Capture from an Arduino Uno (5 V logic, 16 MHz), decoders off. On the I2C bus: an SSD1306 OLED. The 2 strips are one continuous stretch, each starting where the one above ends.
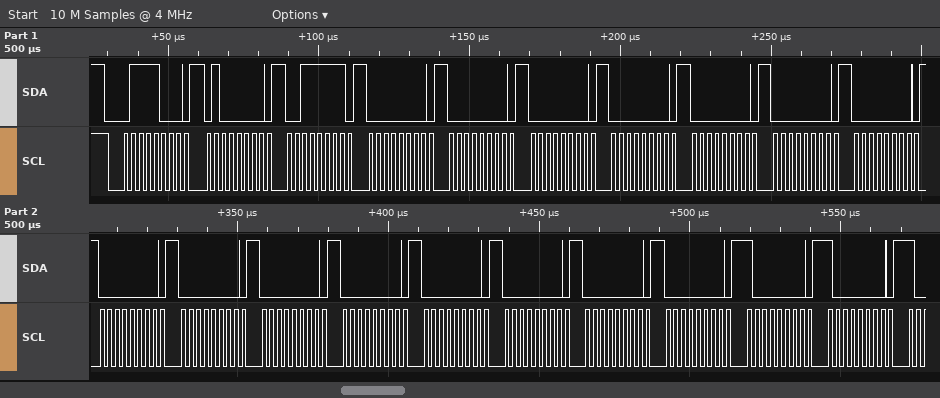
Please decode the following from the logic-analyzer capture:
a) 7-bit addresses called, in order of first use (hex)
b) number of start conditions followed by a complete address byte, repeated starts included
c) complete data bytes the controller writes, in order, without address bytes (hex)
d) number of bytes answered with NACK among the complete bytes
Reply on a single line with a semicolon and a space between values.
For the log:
0x3C; 1; 40 3F 00 00 00 00 00 00 00 00 00 00 00 00 00 00 00 80 80; 0
